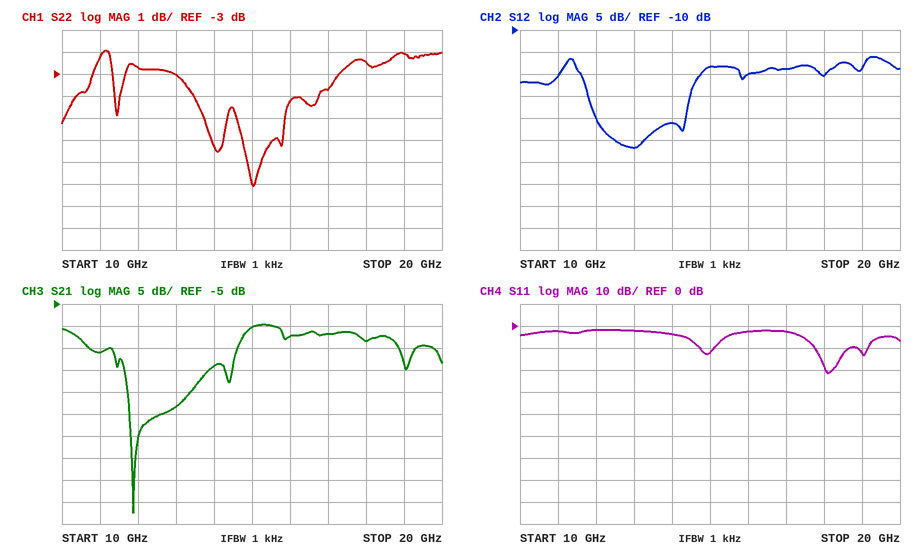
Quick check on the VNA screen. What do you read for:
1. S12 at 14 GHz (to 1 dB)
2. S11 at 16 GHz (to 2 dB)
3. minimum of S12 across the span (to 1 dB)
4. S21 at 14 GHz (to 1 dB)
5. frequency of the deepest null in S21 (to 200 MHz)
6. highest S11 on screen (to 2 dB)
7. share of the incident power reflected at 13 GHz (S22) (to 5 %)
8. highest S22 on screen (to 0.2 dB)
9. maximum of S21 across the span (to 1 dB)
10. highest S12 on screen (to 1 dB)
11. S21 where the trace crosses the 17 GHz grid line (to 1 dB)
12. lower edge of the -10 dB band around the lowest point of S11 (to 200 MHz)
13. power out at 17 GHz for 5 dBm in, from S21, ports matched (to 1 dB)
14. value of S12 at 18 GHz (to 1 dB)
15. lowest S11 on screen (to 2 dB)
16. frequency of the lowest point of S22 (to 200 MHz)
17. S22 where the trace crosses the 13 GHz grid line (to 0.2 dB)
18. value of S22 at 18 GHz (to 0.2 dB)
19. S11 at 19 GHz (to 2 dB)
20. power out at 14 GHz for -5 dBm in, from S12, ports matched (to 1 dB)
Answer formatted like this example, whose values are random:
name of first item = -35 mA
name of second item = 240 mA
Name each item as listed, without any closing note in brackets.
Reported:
S12 at 14 GHz = -31 dB
S11 at 16 GHz = -2 dB
minimum of S12 across the span = -37 dB
S21 at 14 GHz = -19 dB
frequency of the deepest null in S21 = 11.8 GHz
highest S11 on screen = -2 dB
share of the incident power reflected at 13 GHz (S22) = 50 %
highest S22 on screen = -2.0 dB
maximum of S21 across the span = -10 dB
highest S12 on screen = -16 dB
S21 where the trace crosses the 17 GHz grid line = -12 dB
lower edge of the -10 dB band around the lowest point of S11 = 17.8 GHz
power out at 17 GHz for 5 dBm in, from S21, ports matched = -7 dBm
value of S12 at 18 GHz = -20 dB
lowest S11 on screen = -22 dB
frequency of the lowest point of S22 = 15.0 GHz
S22 where the trace crosses the 13 GHz grid line = -3.0 dB
value of S22 at 18 GHz = -2.4 dB
S11 at 19 GHz = -12 dB
power out at 14 GHz for -5 dBm in, from S12, ports matched = -36 dBm
